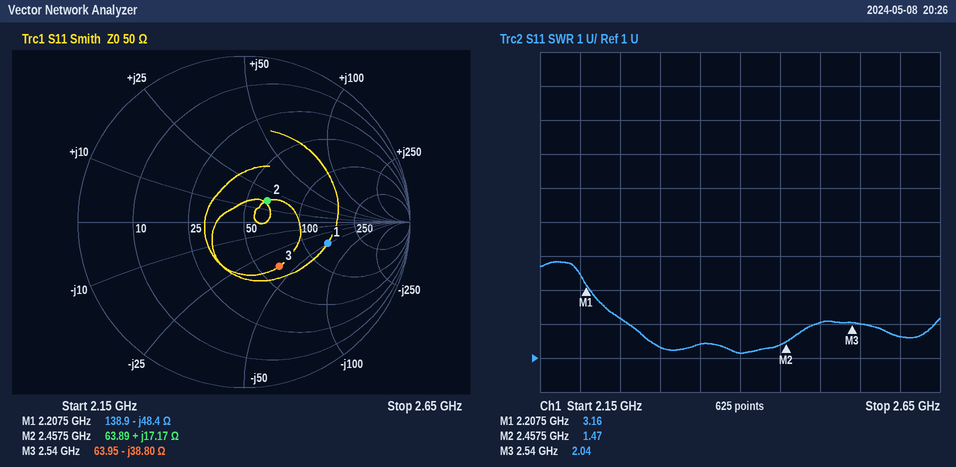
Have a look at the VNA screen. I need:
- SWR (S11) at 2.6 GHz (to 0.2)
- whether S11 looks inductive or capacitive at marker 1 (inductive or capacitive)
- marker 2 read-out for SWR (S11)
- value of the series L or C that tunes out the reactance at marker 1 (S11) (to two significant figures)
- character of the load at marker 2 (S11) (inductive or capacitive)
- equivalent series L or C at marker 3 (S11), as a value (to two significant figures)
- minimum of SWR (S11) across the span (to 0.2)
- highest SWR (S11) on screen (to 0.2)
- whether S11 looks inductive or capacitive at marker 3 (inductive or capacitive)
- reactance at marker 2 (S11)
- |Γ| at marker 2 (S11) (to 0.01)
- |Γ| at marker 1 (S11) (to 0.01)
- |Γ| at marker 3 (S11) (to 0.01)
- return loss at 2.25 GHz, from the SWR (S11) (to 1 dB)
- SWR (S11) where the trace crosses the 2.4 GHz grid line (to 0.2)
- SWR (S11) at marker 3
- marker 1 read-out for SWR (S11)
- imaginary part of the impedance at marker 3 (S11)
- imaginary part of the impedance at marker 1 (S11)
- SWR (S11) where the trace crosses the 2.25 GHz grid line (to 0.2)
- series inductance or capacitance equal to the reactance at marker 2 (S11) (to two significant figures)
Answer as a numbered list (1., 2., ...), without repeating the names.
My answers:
1. 1.6
2. capacitive
3. 1.47
4. 3.5 nH
5. inductive
6. 1.6 pF
7. 1.2
8. 3.8
9. capacitive
10. +17.17 Ω
11. 0.19
12. 0.52
13. 0.34
14. 9 dB
15. 1.2
16. 2.04
17. 3.16
18. -38.80 Ω
19. -48.4 Ω
20. 2.2
21. 1.1 nH
